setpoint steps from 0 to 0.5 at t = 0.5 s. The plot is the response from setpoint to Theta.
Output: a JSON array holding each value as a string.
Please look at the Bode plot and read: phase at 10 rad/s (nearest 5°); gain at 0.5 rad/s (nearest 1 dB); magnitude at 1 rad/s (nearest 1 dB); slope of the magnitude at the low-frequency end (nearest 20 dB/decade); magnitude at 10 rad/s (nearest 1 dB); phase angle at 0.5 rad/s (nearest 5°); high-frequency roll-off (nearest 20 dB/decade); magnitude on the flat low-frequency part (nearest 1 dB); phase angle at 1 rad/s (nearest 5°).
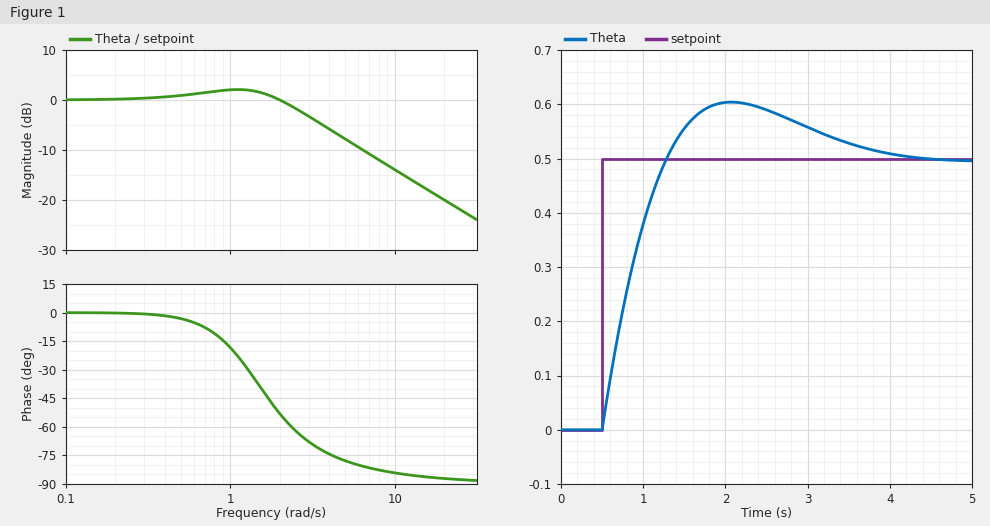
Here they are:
["-85°", "1 dB", "2 dB", "0 dB/decade", "-14 dB", "-5°", "-20 dB/decade", "0 dB", "-20°"]
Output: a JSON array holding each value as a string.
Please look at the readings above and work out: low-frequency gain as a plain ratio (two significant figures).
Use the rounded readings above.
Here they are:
["1.0"]
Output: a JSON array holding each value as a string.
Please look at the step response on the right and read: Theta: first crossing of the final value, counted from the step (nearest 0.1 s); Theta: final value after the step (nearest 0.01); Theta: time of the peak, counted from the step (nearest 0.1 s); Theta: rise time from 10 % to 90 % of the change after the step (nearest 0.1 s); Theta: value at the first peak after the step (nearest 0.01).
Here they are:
["0.8 s", "0.50", "1.6 s", "0.6 s", "0.60"]
